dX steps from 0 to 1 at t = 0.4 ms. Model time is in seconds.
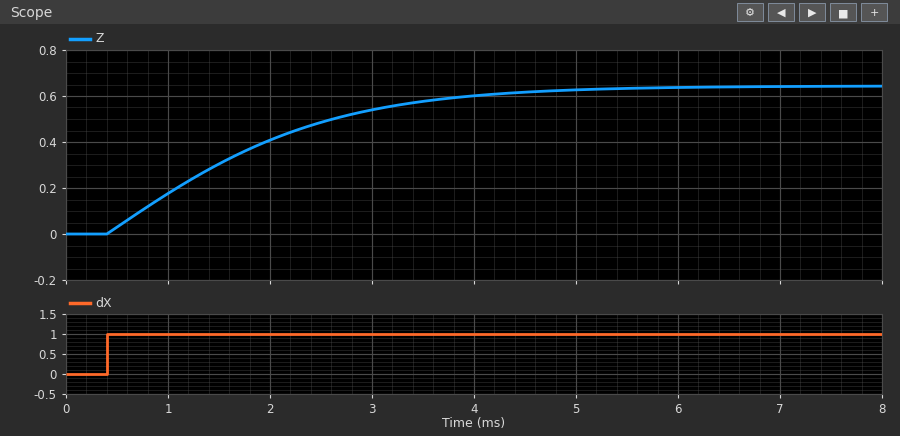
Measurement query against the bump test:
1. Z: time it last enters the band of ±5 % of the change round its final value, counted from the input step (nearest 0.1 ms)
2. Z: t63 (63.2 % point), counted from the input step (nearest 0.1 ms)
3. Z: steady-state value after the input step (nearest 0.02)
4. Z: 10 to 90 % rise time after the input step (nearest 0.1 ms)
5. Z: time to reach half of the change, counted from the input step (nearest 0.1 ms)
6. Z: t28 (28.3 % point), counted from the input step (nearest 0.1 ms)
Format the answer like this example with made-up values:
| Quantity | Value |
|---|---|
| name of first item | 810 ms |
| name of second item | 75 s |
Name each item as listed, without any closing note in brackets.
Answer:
| Quantity | Value |
|---|---|
| Z: time it last enters the band of ±5 % of the change round its final value, counted from the input step | 3.9 ms |
| Z: t63 (63.2 % point), counted from the input step | 1.6 ms |
| Z: steady-state value after the input step | 0.64 |
| Z: 10 to 90 % rise time after the input step | 2.9 ms |
| Z: time to reach half of the change, counted from the input step | 1.2 ms |
| Z: t28 (28.3 % point), counted from the input step | 0.6 ms |
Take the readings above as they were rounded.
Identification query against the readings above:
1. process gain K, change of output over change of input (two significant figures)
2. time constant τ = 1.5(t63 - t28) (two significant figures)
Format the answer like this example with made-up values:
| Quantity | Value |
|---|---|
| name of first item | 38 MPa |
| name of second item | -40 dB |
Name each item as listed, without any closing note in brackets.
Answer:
| Quantity | Value |
|---|---|
| process gain K, change of output over change of input | 0.64 |
| time constant τ = 1.5(t63 - t28) | 1.5 ms |
